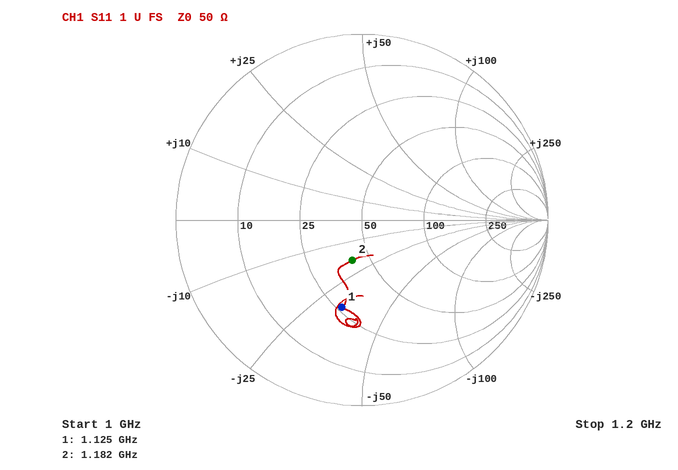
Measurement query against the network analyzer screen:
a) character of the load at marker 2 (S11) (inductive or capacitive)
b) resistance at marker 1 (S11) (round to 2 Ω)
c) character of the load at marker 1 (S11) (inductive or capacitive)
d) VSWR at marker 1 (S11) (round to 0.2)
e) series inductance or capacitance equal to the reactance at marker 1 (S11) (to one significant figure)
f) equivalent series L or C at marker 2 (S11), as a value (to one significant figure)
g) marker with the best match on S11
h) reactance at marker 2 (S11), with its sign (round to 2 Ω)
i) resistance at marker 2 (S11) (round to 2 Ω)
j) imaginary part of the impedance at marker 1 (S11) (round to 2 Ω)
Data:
capacitive
26 Ω
capacitive
2.8
4 pF
7 pF
marker 2
-18 Ω
42 Ω
-32 Ω
